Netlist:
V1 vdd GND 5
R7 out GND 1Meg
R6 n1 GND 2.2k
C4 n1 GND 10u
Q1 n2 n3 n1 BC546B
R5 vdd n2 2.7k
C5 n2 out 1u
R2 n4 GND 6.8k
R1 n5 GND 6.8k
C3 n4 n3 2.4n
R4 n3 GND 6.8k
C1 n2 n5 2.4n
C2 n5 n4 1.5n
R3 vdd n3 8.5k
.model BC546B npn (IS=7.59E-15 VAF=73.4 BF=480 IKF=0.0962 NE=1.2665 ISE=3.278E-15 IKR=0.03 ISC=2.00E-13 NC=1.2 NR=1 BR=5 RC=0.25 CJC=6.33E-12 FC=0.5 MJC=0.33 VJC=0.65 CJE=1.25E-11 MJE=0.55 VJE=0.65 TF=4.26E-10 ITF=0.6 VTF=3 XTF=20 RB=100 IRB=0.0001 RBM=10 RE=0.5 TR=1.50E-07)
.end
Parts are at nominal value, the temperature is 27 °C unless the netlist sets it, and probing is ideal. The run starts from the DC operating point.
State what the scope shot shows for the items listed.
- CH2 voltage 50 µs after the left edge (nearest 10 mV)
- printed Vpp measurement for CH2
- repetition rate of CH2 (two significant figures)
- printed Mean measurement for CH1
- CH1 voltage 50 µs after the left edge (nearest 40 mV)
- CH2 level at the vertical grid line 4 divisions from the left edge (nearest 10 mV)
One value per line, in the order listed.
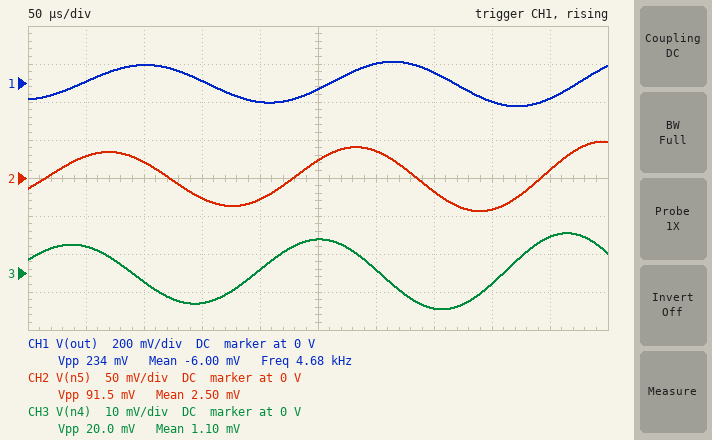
30 mV
91.5 mV
4.7 kHz
-6.00 mV
0 V
-30 mV
